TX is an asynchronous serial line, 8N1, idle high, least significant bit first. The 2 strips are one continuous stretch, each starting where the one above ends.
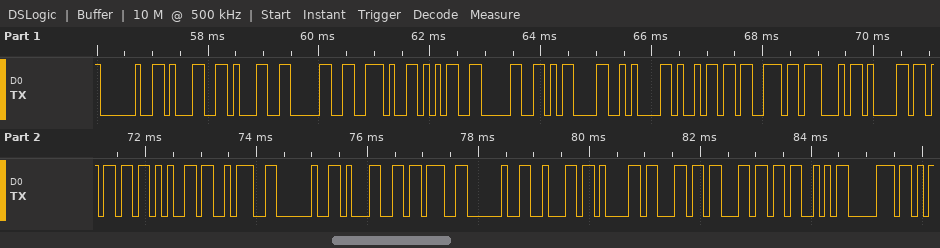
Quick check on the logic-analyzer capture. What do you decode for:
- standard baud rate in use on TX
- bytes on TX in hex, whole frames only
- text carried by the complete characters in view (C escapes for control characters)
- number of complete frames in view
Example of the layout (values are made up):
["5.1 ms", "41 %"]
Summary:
["9600 baud", "20 31 31 30 2E 35 30 0D 0A 69 73 47 61 6D 65 3A 20 31 3B 20 62 61 6C 6C 53 70", "\" 110.50\\r\\nisGame: 1; ballSp\"", "26"]
